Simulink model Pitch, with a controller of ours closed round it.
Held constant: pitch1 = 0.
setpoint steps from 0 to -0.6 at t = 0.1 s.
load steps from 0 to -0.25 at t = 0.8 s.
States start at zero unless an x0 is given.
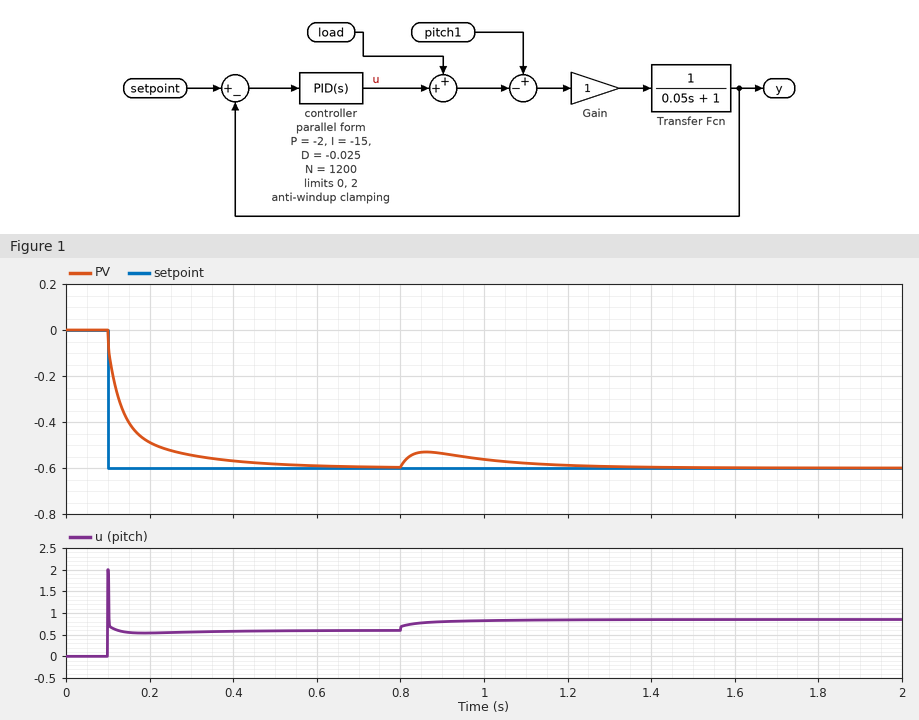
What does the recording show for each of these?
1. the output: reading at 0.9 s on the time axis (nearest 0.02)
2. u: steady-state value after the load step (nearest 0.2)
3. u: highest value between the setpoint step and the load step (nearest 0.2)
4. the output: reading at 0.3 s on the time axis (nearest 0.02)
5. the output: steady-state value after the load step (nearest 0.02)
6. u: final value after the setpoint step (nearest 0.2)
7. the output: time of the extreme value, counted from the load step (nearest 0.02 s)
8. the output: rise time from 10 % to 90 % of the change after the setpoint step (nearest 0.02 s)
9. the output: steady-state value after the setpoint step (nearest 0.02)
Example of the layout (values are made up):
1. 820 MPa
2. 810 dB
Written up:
1. -0.54
2. 0.8
3. 2.0
4. -0.54
5. -0.60
6. 0.6
7. 0.06 s
8. 0.18 s
9. -0.60
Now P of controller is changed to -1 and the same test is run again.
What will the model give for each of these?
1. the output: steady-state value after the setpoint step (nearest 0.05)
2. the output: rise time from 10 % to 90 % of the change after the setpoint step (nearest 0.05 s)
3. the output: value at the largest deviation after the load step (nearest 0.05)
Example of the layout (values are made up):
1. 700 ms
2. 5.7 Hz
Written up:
1. -0.60
2. 0.15 s
3. -0.50
